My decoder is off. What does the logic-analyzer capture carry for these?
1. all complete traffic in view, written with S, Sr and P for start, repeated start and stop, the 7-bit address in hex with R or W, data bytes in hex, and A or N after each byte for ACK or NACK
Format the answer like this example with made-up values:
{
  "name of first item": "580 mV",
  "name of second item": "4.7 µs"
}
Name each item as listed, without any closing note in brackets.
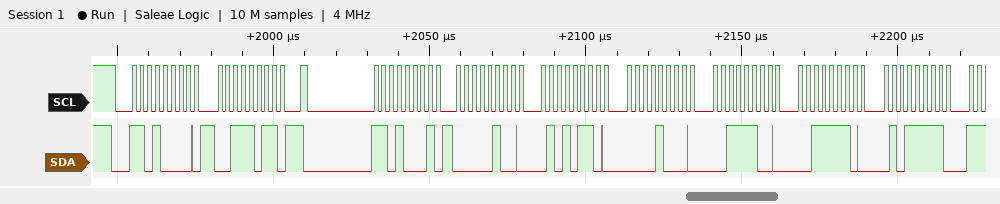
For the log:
{
  "all complete traffic in view, written with S, Sr and P for start, repeated start and stop, the 7-bit address in hex with R or W, data bytes in hex, and A or N after each byte for ACK or NACK": "S 68W A 3B A Sr 68R A 04 A 56 A 08 A 3C A 3E A 5F A"
}
